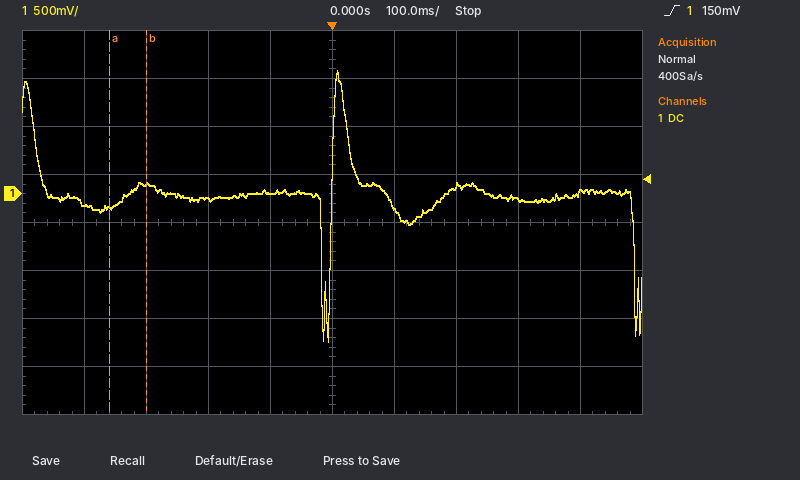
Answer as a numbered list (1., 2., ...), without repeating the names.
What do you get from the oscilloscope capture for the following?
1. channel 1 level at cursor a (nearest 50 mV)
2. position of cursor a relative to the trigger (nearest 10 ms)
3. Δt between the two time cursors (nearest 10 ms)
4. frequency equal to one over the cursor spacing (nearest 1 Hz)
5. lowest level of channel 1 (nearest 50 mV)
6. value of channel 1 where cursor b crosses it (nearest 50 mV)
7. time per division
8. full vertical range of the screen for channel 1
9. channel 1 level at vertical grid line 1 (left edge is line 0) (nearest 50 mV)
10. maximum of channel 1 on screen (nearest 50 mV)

1. -150 mV
2. -360 ms
3. 60 ms
4. 17 Hz
5. -1.55 V
6. 100 mV
7. 100 ms
8. 4 V
9. -100 mV
10. 1.30 V
